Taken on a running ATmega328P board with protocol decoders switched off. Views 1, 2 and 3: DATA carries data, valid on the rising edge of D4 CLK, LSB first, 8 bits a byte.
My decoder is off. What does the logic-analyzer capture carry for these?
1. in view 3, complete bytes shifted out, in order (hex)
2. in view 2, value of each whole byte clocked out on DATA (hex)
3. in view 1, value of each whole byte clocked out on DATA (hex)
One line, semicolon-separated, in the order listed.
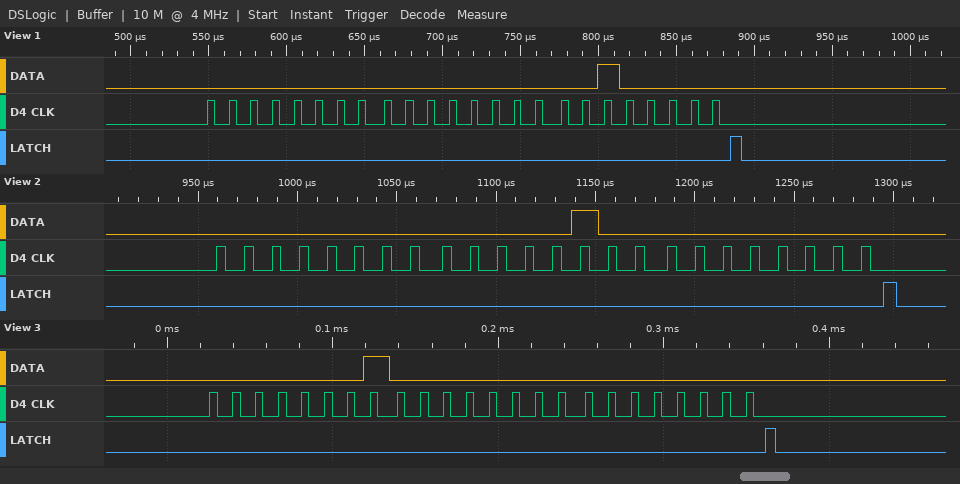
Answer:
0x80 0x00 0x00; 00 20 00; 00 00 04
